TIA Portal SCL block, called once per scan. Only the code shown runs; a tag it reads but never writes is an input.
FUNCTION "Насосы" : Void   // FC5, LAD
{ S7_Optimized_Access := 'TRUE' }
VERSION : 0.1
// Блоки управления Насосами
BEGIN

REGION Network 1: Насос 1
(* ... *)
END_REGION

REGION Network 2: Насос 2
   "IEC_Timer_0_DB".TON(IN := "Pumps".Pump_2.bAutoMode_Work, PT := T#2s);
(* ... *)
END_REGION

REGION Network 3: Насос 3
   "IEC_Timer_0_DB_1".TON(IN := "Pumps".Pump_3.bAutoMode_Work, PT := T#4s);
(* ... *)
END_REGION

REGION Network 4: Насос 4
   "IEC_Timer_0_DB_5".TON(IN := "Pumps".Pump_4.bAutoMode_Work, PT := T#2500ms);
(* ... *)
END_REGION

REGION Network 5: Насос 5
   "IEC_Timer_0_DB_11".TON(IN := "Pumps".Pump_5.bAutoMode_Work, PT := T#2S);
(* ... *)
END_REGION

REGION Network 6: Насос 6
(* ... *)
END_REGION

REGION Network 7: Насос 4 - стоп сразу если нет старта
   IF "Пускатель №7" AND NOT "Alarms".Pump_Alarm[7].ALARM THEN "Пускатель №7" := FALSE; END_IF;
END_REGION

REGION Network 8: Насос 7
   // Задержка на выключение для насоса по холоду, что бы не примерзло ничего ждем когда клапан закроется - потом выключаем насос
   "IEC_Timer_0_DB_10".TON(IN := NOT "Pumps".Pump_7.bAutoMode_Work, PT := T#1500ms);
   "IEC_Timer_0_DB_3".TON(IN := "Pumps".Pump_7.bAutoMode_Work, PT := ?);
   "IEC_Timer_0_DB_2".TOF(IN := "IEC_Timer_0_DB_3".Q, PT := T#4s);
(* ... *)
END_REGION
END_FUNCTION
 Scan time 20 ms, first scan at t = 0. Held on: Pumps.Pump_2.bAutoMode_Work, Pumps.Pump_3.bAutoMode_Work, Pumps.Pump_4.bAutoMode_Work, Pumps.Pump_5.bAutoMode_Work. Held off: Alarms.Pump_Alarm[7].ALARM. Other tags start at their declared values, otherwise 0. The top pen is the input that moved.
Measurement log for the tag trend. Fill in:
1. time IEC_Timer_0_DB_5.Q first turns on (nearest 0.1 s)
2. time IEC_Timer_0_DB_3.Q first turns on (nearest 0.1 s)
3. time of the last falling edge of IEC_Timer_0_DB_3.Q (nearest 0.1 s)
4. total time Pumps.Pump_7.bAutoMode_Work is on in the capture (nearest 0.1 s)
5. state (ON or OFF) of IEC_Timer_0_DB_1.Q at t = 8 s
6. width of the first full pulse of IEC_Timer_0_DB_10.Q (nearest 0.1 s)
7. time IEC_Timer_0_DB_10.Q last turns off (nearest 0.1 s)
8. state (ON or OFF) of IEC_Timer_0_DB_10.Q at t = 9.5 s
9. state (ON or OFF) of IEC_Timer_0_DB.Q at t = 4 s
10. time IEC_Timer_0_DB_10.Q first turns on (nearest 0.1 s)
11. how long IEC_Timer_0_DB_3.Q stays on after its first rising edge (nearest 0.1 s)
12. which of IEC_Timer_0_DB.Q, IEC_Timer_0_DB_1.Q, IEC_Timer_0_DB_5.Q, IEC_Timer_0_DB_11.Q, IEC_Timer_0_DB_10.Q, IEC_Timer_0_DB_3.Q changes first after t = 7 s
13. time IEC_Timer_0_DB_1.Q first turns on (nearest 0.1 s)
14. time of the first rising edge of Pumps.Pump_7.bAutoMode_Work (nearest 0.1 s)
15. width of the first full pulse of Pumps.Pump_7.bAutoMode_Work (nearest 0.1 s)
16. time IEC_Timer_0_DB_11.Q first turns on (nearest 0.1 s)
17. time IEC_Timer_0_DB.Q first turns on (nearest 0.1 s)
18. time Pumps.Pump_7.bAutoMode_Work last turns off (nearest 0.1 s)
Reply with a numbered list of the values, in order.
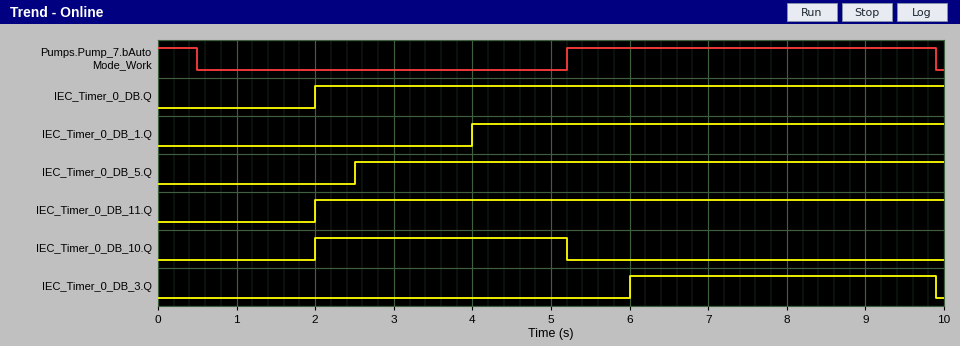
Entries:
1. 2.5 s
2. 6.0 s
3. 9.9 s
4. 5.2 s
5. ON
6. 3.2 s
7. 5.2 s
8. OFF
9. ON
10. 2.0 s
11. 3.9 s
12. IEC_Timer_0_DB_3.Q
13. 4.0 s
14. 5.2 s
15. 4.7 s
16. 2.0 s
17. 2.0 s
18. 9.9 s
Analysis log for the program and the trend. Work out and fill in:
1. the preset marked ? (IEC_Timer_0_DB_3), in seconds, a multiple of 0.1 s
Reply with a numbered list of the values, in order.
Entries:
1. 0.8 s
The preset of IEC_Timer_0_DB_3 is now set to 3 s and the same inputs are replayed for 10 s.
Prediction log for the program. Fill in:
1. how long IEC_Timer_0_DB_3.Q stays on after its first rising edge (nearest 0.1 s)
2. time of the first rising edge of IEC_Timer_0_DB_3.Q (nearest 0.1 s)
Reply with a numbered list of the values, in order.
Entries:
1. 1.7 s
2. 8.2 s
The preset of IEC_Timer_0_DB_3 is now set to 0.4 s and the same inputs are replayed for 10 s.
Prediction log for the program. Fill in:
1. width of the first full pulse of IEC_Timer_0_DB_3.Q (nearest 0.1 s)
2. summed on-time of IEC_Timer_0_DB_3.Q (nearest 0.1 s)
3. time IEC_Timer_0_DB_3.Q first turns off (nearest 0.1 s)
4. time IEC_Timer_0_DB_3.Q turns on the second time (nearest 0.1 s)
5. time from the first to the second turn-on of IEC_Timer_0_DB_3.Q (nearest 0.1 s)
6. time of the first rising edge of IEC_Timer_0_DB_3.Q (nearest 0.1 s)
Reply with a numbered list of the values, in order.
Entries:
1. 0.1 s
2. 4.4 s
3. 0.5 s
4. 5.6 s
5. 5.2 s
6. 0.4 s
